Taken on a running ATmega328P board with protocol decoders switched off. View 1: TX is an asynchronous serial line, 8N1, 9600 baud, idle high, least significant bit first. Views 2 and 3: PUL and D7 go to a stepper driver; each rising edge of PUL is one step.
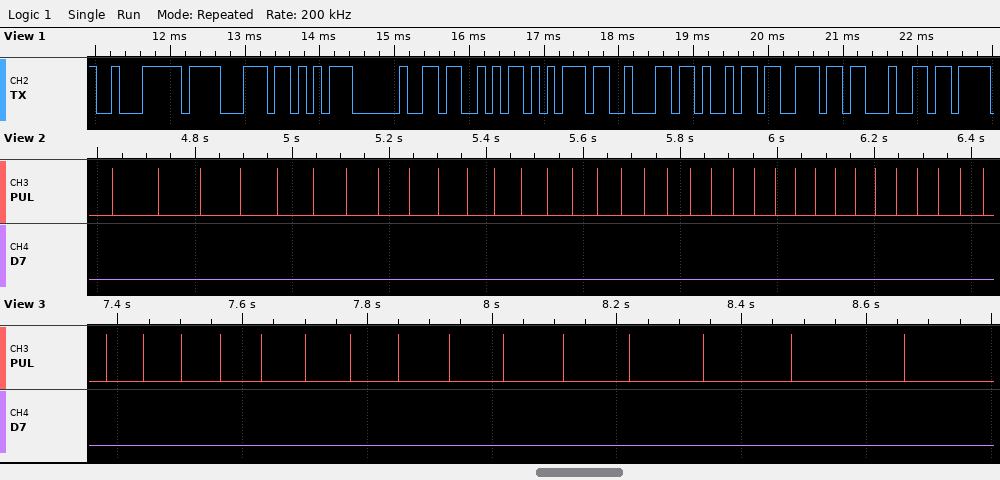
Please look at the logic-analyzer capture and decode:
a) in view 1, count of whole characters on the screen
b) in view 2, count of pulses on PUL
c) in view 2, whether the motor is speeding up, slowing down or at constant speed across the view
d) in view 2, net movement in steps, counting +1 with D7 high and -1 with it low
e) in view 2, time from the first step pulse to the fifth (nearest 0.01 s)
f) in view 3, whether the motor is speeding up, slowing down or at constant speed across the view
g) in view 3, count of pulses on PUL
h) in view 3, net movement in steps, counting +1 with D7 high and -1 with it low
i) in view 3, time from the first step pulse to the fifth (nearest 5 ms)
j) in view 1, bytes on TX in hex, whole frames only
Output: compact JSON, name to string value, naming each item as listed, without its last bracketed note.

{"in view 1, count of whole characters on the screen": "10", "in view 2, count of pulses on PUL": "34", "in view 2, whether the motor is speeding up, slowing down or at constant speed across the view": "speeding up", "in view 2, net movement in steps, counting +1 with D7 high and -1 with it low": "-34", "in view 2, time from the first step pulse to the fifth": "0.34 s", "in view 3, whether the motor is speeding up, slowing down or at constant speed across the view": "slowing down", "in view 3, count of pulses on PUL": "15", "in view 3, net movement in steps, counting +1 with D7 high and -1 with it low": "-15", "in view 3, time from the first step pulse to the fifth": "250 ms", "in view 1, bytes on TX in hex, whole frames only": "E2 8F AB 20 53 75 62 69 6E 64"}
